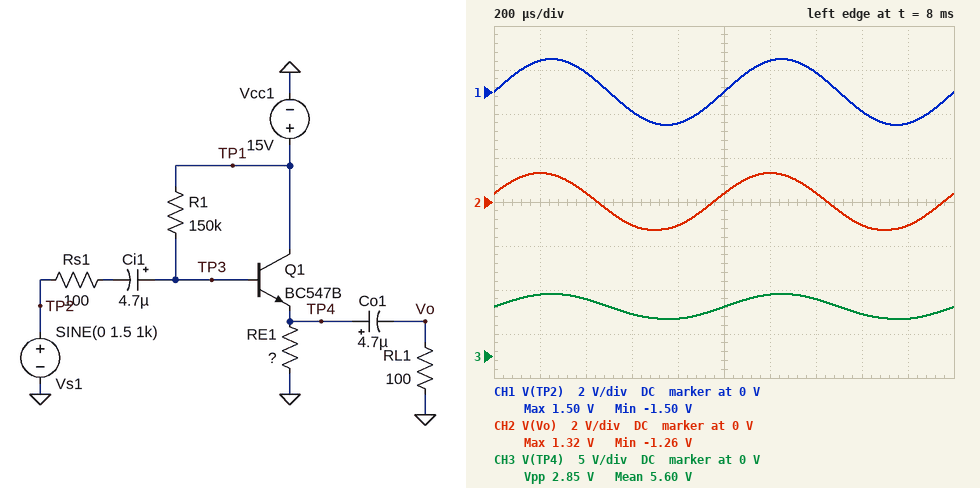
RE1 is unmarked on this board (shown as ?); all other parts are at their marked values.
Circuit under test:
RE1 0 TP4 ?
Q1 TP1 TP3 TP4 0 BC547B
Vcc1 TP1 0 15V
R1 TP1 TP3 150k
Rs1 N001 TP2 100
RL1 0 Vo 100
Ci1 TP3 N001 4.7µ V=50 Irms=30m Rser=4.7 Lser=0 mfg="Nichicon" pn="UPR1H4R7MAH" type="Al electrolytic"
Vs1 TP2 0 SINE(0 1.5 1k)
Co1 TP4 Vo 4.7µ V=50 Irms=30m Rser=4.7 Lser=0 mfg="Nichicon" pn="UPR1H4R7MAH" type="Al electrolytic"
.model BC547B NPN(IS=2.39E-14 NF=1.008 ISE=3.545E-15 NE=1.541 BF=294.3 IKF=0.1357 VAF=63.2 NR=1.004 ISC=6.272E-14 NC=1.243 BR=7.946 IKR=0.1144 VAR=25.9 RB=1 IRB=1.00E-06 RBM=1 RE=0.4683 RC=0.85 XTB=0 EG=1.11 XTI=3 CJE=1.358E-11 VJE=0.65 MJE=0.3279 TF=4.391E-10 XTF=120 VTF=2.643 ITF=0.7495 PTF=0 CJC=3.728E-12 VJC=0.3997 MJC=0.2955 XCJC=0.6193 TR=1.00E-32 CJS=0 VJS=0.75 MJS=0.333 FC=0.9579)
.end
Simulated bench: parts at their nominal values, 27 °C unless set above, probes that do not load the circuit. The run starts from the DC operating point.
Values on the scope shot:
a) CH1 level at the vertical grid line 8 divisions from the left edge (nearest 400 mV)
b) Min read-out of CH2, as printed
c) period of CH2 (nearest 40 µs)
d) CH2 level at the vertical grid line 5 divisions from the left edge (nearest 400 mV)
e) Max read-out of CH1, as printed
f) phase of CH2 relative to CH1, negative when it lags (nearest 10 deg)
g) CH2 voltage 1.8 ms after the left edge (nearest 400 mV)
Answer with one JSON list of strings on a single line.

["-800 mV", "-1.26 V", "1.00 ms", "400 mV", "1.50 V", "20 deg", "-1.2 V"]
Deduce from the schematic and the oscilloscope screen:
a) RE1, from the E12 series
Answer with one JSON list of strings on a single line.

["330 Ω"]
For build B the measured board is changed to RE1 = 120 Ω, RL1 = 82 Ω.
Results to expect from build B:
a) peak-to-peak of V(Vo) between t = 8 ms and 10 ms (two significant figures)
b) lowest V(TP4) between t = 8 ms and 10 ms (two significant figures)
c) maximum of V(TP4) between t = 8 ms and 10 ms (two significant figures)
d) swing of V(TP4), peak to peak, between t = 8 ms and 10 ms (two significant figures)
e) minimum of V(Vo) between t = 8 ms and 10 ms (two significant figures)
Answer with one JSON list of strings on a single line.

["2.4 V", "1.4 V", "4.2 V", "2.7 V", "-1.1 V"]
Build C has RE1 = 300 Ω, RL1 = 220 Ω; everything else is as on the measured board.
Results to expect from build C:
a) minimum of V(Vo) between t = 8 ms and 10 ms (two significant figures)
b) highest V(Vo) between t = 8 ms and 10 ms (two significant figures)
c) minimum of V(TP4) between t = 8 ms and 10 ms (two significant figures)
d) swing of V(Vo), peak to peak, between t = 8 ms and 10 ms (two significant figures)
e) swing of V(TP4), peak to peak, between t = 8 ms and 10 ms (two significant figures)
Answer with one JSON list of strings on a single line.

["-1.4 V", "1.4 V", "3.8 V", "2.8 V", "2.9 V"]
